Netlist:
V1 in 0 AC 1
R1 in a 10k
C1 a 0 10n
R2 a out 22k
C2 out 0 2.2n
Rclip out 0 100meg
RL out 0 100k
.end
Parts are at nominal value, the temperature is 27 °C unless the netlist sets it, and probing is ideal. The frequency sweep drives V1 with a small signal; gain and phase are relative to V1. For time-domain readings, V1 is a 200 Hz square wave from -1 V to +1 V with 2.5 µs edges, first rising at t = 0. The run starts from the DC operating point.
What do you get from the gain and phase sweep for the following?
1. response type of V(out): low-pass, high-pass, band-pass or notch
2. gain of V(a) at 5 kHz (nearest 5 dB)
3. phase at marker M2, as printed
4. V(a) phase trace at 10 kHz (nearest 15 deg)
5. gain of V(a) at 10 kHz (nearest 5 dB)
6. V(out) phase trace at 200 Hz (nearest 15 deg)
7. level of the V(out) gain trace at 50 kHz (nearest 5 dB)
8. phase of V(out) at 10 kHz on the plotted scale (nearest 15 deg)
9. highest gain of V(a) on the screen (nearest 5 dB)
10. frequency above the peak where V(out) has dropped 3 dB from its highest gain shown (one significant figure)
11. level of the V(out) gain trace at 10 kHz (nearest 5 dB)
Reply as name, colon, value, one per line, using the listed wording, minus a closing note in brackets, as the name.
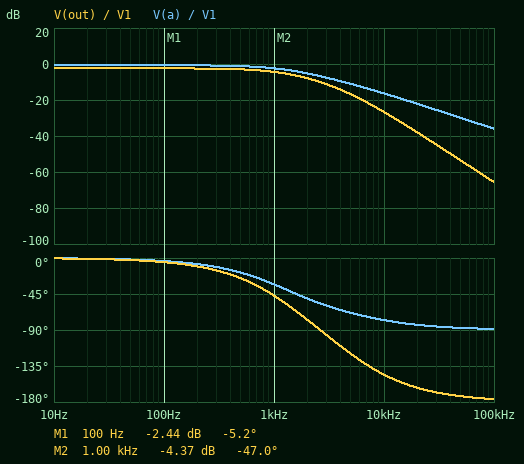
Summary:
response type of V(out): low-pass, high-pass, band-pass or notch: low-pass
gain of V(a) at 5 kHz: -10 dB
phase at marker M2, as printed: -47.0 deg
V(a) phase trace at 10 kHz: -75 deg
gain of V(a) at 10 kHz: -15 dB
V(out) phase trace at 200 Hz: -15 deg
level of the V(out) gain trace at 50 kHz: -55 dB
phase of V(out) at 10 kHz on the plotted scale: -150 deg
highest gain of V(a) on the screen: 0 dB
frequency above the peak where V(out) has dropped 3 dB from its highest gain shown: 1 kHz
level of the V(out) gain trace at 10 kHz: -25 dB
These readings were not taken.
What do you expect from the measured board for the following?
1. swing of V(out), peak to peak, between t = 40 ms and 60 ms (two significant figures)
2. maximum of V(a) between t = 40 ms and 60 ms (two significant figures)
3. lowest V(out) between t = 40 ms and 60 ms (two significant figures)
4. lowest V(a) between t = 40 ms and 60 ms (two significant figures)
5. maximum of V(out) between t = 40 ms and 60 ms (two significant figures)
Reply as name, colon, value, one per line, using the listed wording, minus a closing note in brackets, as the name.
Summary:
swing of V(out), peak to peak, between t = 40 ms and 60 ms: 1.5 V
maximum of V(a) between t = 40 ms and 60 ms: 920 mV
lowest V(out) between t = 40 ms and 60 ms: -760 mV
lowest V(a) between t = 40 ms and 60 ms: -920 mV
maximum of V(out) between t = 40 ms and 60 ms: 760 mV
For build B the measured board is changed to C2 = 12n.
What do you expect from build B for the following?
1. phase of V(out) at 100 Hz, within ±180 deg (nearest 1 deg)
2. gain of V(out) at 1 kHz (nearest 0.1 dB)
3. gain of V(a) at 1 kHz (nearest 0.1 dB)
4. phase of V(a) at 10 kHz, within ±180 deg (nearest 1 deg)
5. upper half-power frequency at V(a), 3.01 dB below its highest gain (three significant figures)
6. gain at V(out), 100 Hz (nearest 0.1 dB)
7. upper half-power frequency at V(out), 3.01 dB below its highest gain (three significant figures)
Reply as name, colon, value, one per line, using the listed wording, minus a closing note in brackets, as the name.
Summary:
phase of V(out) at 100 Hz, within ±180 deg: -14 deg
gain of V(out) at 1 kHz: -10.1 dB
gain of V(a) at 1 kHz: -3.8 dB
phase of V(a) at 10 kHz, within ±180 deg: -77 deg
upper half-power frequency at V(a), 3.01 dB below its highest gain: 956 Hz
gain at V(out), 100 Hz: -2.6 dB
upper half-power frequency at V(out), 3.01 dB below its highest gain: 479 Hz
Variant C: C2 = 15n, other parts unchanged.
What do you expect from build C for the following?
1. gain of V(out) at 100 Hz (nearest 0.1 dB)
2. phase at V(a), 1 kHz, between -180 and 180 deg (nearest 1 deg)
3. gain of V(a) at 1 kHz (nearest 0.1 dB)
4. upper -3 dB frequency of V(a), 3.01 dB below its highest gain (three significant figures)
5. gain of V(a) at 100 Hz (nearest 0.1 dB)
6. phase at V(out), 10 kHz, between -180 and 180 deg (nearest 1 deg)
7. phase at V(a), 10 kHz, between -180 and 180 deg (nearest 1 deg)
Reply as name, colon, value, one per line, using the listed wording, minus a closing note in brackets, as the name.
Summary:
gain of V(out) at 100 Hz: -2.7 dB
phase at V(a), 1 kHz, between -180 and 180 deg: -30 deg
gain of V(a) at 1 kHz: -3.9 dB
upper -3 dB frequency of V(a), 3.01 dB below its highest gain: 897 Hz
gain of V(a) at 100 Hz: -0.8 dB
phase at V(out), 10 kHz, between -180 and 180 deg: -164 deg
phase at V(a), 10 kHz, between -180 and 180 deg: -77 deg
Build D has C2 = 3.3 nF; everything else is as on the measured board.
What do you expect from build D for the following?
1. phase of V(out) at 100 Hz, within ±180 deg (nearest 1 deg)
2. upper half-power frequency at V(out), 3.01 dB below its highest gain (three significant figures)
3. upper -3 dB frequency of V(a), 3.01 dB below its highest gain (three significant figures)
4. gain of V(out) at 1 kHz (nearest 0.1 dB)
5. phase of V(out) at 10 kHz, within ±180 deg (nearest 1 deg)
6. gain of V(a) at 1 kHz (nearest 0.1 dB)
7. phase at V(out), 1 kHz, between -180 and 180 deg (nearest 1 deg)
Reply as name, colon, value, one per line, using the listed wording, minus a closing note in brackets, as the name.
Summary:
phase of V(out) at 100 Hz, within ±180 deg: -6 deg
upper half-power frequency at V(out), 3.01 dB below its highest gain: 1.12 kHz
upper -3 dB frequency of V(a), 3.01 dB below its highest gain: 1.35 kHz
gain of V(out) at 1 kHz: -4.9 dB
phase of V(out) at 10 kHz, within ±180 deg: -152 deg
gain of V(a) at 1 kHz: -2.6 dB
phase at V(out), 1 kHz, between -180 and 180 deg: -54 deg
